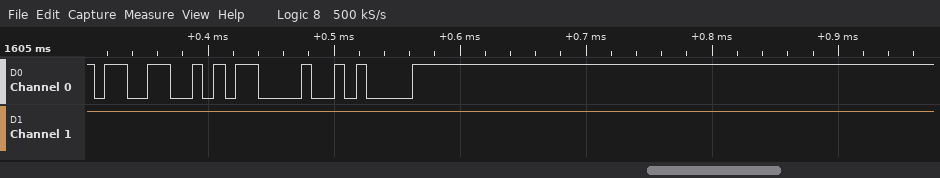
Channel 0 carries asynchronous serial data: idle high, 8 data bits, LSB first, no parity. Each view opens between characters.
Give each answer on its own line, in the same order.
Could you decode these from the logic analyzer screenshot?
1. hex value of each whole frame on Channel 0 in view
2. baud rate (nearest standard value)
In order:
33, 0D, 0A
115200 baud
